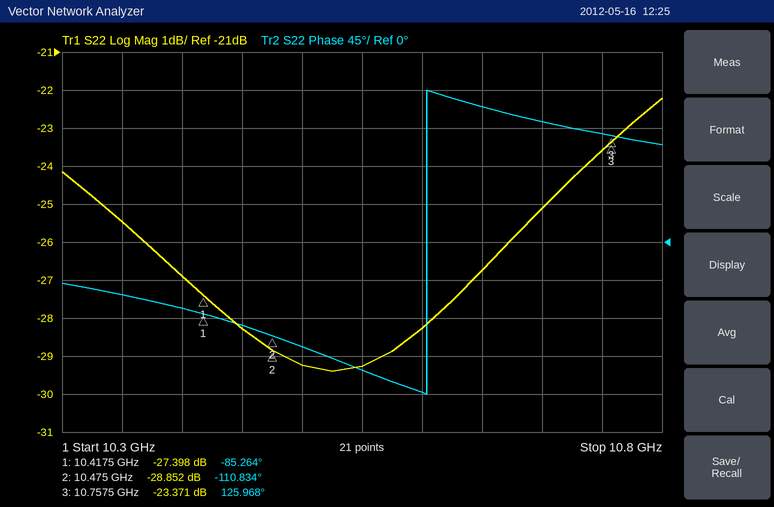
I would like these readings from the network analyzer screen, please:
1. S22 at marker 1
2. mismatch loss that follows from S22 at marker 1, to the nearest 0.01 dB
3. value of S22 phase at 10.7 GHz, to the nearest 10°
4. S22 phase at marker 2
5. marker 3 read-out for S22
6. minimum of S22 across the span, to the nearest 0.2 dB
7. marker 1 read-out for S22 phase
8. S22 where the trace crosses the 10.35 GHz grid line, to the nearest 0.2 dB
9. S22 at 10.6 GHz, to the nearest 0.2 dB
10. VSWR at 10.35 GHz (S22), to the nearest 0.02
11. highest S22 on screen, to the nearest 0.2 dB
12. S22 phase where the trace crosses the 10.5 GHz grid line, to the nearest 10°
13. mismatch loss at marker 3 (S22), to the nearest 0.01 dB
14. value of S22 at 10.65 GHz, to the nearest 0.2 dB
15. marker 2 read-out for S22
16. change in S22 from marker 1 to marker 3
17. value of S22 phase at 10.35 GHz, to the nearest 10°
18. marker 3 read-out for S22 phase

-27.398 dB
0.01 dB
140°
-110.834°
-23.371 dB
-29.4 dB
-85.264°
-25.4 dB
-28.2 dB
1.12
-22.2 dB
-120°
0.02 dB
-26.8 dB
-28.852 dB
4.027 dB
-60°
125.968°
